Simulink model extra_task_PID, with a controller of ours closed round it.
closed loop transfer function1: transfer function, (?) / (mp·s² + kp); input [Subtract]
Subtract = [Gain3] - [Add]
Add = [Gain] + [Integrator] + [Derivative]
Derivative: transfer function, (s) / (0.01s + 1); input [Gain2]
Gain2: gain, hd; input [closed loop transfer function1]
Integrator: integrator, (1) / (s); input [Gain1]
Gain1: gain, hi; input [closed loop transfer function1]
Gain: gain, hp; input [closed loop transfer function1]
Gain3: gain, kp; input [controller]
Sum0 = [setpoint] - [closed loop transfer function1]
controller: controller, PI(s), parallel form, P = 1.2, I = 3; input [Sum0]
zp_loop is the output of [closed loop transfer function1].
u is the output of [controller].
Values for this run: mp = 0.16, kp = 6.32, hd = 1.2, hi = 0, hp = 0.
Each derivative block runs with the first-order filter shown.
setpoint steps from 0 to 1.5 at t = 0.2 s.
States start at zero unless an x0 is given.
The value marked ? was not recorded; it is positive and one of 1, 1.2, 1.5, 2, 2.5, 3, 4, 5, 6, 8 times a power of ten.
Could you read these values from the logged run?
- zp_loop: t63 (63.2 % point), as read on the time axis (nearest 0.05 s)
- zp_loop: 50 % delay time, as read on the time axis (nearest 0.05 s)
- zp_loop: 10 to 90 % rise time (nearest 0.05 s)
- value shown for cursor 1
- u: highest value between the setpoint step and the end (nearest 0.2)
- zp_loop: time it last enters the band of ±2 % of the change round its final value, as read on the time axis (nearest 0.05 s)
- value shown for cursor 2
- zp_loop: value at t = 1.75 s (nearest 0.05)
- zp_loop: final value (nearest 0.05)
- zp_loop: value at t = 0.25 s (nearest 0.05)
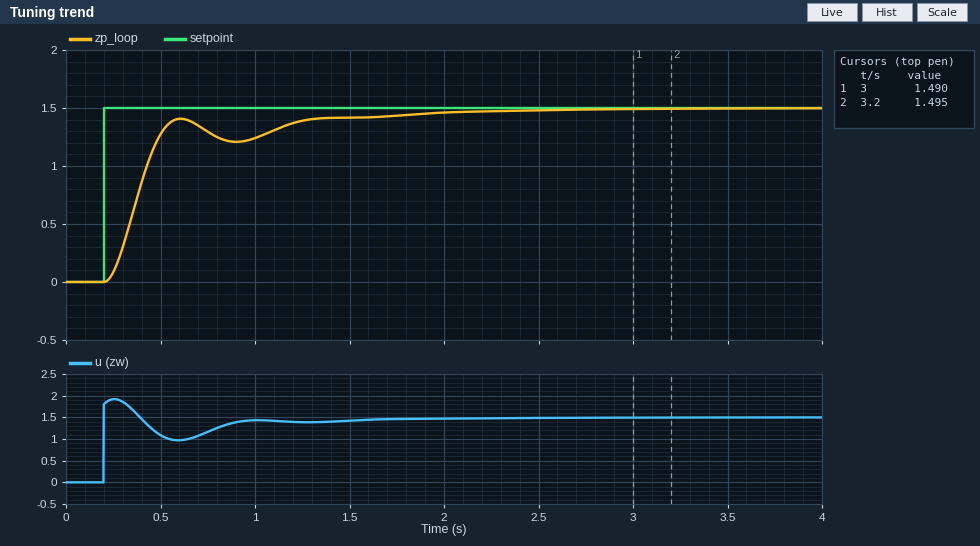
0.40 s
0.40 s
0.25 s
1.490
2.0
2.20 s
1.495
1.45
1.50
0.10
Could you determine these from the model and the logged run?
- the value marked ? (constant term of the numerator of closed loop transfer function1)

1
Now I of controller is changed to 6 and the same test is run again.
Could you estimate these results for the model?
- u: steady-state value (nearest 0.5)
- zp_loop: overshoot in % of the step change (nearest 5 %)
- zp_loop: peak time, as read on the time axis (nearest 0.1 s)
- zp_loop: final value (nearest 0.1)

1.5
15 %
0.6 s
1.5
